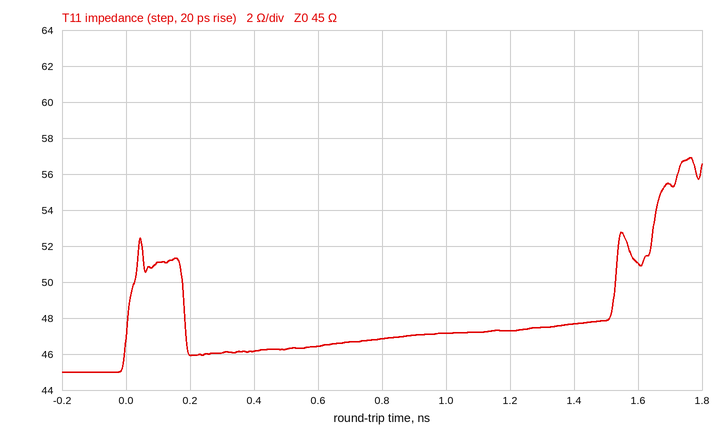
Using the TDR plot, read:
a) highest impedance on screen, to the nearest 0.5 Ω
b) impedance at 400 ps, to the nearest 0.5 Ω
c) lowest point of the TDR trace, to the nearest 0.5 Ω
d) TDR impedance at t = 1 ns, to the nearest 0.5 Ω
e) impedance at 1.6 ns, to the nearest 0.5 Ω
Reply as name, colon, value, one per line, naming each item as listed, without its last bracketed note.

highest impedance on screen, to the nearest 0.5 Ω: 57.0 Ω
impedance at 400 ps, to the nearest 0.5 Ω: 46.0 Ω
lowest point of the TDR trace, to the nearest 0.5 Ω: 45.0 Ω
TDR impedance at t = 1 ns, to the nearest 0.5 Ω: 47.0 Ω
impedance at 1.6 ns, to the nearest 0.5 Ω: 51.0 Ω
